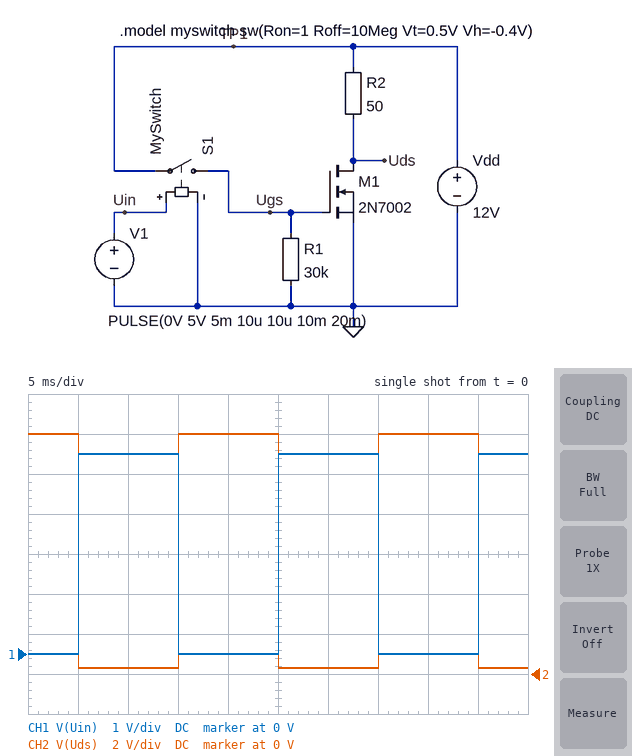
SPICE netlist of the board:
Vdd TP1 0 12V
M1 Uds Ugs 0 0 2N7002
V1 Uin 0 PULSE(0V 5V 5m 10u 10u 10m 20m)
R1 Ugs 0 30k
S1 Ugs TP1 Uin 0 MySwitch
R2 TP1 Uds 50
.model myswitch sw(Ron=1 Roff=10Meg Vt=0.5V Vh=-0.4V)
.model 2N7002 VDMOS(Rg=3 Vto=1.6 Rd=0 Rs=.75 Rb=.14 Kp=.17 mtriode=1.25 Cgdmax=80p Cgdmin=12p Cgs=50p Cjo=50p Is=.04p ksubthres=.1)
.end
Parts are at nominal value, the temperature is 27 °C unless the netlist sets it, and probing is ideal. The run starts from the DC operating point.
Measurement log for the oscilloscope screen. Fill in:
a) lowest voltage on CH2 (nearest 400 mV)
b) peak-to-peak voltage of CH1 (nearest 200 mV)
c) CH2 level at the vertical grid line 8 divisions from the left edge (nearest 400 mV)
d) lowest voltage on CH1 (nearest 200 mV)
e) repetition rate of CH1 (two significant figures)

400 mV
5.0 V
12.0 V
0 V
50 Hz
